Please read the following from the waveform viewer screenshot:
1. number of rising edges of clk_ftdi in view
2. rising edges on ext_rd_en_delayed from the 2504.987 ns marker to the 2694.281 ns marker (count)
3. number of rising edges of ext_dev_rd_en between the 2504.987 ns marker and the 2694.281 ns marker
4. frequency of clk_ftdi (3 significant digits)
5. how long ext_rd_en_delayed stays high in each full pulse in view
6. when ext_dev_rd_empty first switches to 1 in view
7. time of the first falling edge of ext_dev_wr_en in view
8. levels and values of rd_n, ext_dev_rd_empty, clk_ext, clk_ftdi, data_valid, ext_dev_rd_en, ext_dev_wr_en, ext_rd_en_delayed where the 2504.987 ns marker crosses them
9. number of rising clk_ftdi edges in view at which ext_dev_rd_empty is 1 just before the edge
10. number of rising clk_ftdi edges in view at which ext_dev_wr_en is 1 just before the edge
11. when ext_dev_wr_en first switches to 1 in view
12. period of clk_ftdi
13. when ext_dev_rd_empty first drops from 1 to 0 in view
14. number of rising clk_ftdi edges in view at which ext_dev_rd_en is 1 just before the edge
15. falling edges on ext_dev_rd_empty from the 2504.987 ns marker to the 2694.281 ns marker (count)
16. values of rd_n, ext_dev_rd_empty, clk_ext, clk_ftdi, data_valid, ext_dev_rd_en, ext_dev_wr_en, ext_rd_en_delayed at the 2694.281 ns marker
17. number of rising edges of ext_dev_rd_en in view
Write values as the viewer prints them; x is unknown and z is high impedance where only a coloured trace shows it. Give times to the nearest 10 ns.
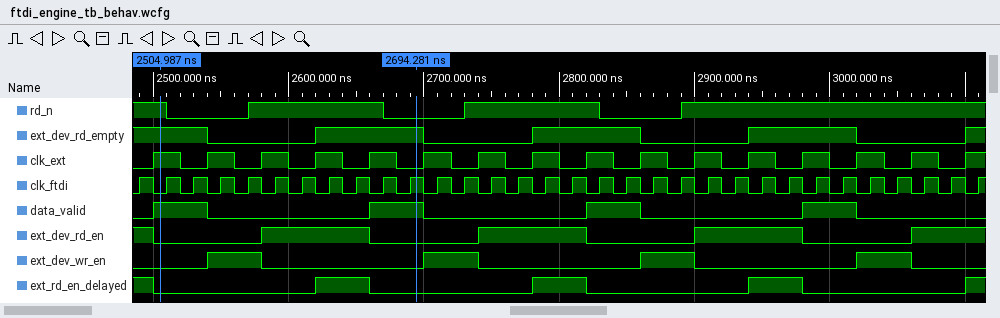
32
1
1
50.0 MHz
40 ns, 40 ns, 40 ns
2620 ns
2580 ns
rd_n=1, ext_dev_rd_empty=1, clk_ext=1, clk_ftdi=0, data_valid=1, ext_dev_rd_en=0, ext_dev_wr_en=0, ext_rd_en_delayed=0
16
8
2540 ns
20 ns
2540 ns
16
1
rd_n=0, ext_dev_rd_empty=1, clk_ext=0, clk_ftdi=1, data_valid=1, ext_dev_rd_en=0, ext_dev_wr_en=0, ext_rd_en_delayed=0
4
